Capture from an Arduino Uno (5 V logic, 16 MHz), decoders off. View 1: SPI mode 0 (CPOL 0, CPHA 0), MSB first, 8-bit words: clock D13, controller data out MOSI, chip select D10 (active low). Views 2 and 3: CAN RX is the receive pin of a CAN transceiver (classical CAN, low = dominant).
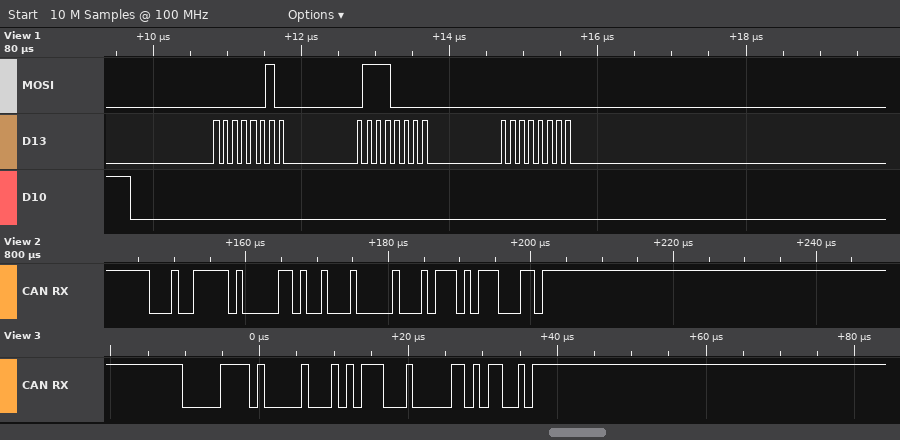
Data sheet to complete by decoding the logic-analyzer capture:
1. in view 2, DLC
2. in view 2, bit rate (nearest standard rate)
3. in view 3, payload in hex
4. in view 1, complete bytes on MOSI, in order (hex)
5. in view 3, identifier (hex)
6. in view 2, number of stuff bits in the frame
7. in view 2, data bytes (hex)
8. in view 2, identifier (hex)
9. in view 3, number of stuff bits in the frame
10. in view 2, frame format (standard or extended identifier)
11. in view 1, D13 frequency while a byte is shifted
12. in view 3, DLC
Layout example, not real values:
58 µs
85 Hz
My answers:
2
1000 kbit/s
5C
0x02 0x70 0x00
0x074
3
91 00
0x13F
3
standard
8 MHz
1
